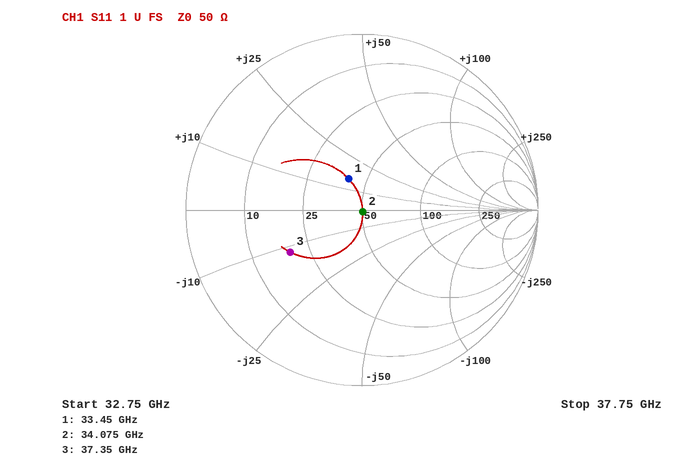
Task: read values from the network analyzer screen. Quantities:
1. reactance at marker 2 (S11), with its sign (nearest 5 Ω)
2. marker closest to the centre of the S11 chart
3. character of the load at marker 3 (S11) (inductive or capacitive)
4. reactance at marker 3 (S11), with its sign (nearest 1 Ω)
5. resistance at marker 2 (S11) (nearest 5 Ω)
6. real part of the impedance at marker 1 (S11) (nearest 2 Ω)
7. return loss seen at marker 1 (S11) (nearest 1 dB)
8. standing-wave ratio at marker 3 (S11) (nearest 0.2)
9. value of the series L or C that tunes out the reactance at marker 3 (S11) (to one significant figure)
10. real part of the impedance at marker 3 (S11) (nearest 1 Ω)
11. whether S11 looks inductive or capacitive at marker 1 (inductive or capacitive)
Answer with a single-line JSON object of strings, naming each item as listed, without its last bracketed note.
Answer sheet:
{"reactance at marker 2 (S11), with its sign": "0 Ω", "marker closest to the centre of the S11 chart": "marker 2", "character of the load at marker 3 (S11)": "capacitive", "reactance at marker 3 (S11), with its sign": "-12 Ω", "resistance at marker 2 (S11)": "50 Ω", "real part of the impedance at marker 1 (S11)": "40 Ω", "return loss seen at marker 1 (S11)": "14 dB", "standing-wave ratio at marker 3 (S11)": "2.8", "value of the series L or C that tunes out the reactance at marker 3 (S11)": "50 pH", "real part of the impedance at marker 3 (S11)": "19 Ω", "whether S11 looks inductive or capacitive at marker 1": "inductive"}
